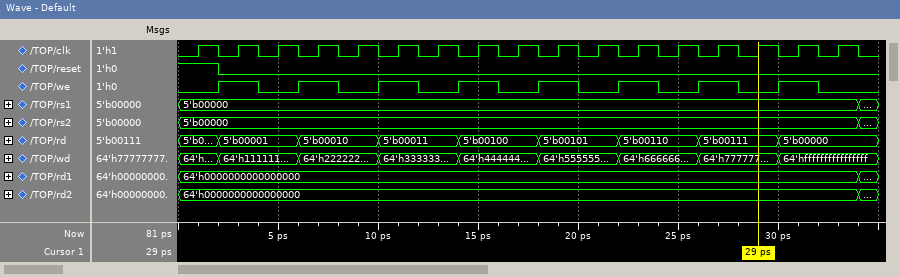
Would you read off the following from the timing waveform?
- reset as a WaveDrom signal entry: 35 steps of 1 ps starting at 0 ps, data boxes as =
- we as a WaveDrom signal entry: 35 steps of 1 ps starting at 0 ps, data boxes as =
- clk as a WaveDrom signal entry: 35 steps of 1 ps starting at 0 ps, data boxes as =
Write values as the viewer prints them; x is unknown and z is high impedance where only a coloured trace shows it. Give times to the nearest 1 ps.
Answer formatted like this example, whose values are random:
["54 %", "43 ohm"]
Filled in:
["{name: 'reset', wave: '1.0................................'}", "{name: 'we', wave: '0.1.0.1.0.1.0.1.0.1.0.1.0.1.0.1.0..'}", "{name: 'clk', wave: '01010101010101010101010101010101010'}"]
